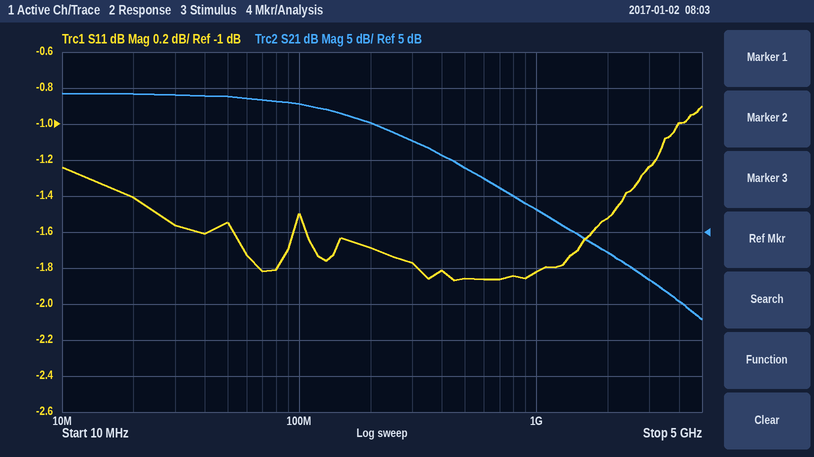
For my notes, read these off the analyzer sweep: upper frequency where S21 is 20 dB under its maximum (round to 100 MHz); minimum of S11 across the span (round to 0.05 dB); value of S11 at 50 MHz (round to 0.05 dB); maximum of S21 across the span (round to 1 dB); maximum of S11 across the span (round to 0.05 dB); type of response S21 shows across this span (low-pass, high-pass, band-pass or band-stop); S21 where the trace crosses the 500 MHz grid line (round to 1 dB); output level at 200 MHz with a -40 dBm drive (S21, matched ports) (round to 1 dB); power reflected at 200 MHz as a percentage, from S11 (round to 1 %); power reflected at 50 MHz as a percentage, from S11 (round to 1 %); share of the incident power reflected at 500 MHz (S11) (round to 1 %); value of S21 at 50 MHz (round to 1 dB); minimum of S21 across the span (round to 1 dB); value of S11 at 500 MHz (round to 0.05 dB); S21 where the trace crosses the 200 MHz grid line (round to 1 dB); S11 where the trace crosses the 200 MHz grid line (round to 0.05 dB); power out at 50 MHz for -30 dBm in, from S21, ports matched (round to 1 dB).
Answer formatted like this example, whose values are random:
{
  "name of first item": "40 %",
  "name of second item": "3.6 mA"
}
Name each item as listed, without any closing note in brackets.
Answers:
{
  "upper frequency where S21 is 20 dB under its maximum": "1.6 GHz",
  "minimum of S11 across the span": "-1.85 dB",
  "value of S11 at 50 MHz": "-1.55 dB",
  "maximum of S21 across the span": "24 dB",
  "maximum of S11 across the span": "-0.90 dB",
  "type of response S21 shows across this span": "low-pass",
  "S21 where the trace crosses the 500 MHz grid line": "14 dB",
  "output level at 200 MHz with a -40 dBm drive (S21, matched ports)": "-20 dBm",
  "power reflected at 200 MHz as a percentage, from S11": "68 %",
  "power reflected at 50 MHz as a percentage, from S11": "70 %",
  "share of the incident power reflected at 500 MHz (S11)": "65 %",
  "value of S21 at 50 MHz": "24 dB",
  "minimum of S21 across the span": "-7 dB",
  "value of S11 at 500 MHz": "-1.85 dB",
  "S21 where the trace crosses the 200 MHz grid line": "20 dB",
  "S11 where the trace crosses the 200 MHz grid line": "-1.70 dB",
  "power out at 50 MHz for -30 dBm in, from S21, ports matched": "-6 dBm"
}
